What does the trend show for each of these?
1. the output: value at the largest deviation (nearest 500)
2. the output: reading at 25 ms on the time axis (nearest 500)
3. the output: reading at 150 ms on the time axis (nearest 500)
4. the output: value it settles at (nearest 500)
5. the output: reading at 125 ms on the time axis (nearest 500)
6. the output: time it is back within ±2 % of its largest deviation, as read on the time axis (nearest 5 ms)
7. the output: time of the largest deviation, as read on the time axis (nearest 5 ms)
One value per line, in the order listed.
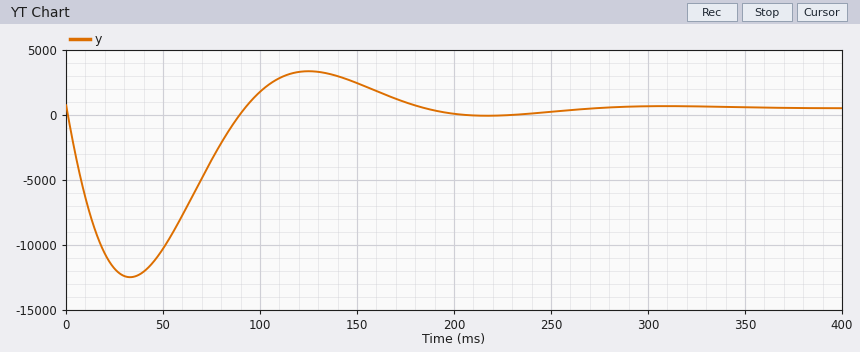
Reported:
-12500
-12000
2500
500
3500
255 ms
35 ms
